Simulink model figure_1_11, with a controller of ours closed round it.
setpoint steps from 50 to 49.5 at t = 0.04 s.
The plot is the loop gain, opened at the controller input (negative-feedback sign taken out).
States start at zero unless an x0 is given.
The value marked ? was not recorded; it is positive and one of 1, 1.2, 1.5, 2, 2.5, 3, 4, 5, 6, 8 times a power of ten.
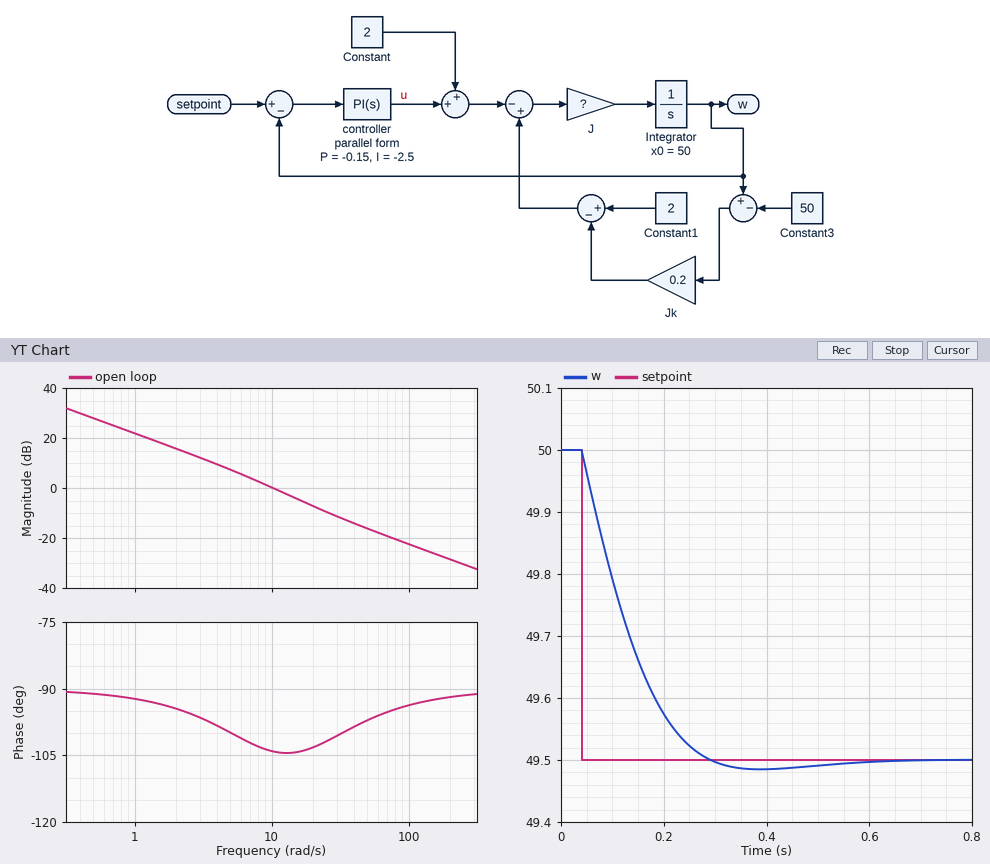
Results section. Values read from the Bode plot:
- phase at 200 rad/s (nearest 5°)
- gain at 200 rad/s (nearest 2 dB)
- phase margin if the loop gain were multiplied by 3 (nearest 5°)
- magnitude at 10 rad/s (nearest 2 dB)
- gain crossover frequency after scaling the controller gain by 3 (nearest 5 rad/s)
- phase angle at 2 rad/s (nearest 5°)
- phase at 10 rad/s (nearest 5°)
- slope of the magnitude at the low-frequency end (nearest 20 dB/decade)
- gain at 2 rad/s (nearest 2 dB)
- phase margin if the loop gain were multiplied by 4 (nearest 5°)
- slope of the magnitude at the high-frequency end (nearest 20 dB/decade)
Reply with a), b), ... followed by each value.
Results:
a) -90°
b) -28 dB
c) 80°
d) 0 dB
e) 25 rad/s
f) -95°
g) -105°
h) -20 dB/decade
i) 16 dB
j) 80°
k) -20 dB/decade
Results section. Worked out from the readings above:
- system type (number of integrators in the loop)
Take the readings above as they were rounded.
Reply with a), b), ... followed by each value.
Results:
a) 1
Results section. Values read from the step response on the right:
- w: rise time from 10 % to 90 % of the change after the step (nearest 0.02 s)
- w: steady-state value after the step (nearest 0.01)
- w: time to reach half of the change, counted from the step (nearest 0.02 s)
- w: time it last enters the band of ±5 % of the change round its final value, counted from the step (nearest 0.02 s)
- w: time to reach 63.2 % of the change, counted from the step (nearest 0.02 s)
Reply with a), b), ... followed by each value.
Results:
a) 0.16 s
b) 49.50
c) 0.08 s
d) 0.20 s
e) 0.10 s
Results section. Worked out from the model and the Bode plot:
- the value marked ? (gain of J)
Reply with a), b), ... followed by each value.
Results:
a) 50
